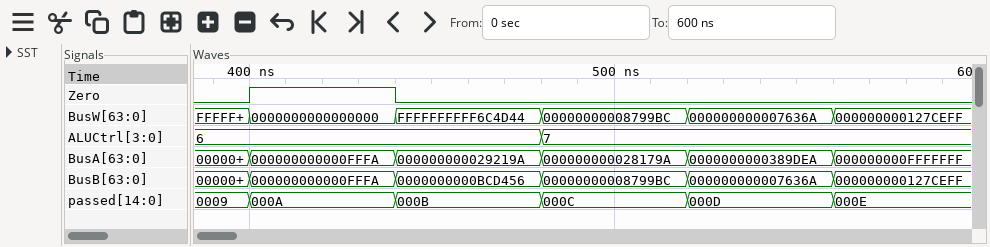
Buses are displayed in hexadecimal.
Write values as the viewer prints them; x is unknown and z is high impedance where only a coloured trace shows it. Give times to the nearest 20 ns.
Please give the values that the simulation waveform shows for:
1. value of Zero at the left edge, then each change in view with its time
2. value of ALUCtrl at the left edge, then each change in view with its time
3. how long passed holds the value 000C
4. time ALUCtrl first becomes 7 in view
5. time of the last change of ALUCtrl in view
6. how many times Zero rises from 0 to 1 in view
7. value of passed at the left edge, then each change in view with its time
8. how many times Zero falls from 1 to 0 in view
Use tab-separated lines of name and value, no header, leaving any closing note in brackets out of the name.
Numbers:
value of Zero at the left edge, then each change in view with its time	0, 1 at 400 ns, 0 at 440 ns
value of ALUCtrl at the left edge, then each change in view with its time	6, 7 at 480 ns
how long passed holds the value 000C	40 ns
time ALUCtrl first becomes 7 in view	480 ns
time of the last change of ALUCtrl in view	480 ns
how many times Zero rises from 0 to 1 in view	1
value of passed at the left edge, then each change in view with its time	0009, 000A at 400 ns, 000B at 440 ns, 000C at 480 ns, 000D at 520 ns, 000E at 560 ns
how many times Zero falls from 1 to 0 in view	1
